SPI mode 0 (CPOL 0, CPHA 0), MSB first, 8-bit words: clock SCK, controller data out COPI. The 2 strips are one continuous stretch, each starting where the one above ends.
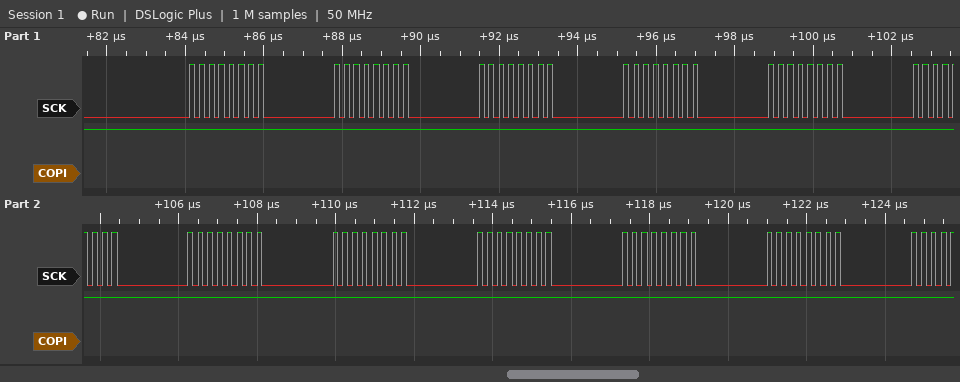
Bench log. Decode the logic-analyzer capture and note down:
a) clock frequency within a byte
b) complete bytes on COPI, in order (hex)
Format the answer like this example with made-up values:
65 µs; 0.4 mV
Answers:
4 MHz; FF FF FF FF FF FF FF FF FF FF FF
